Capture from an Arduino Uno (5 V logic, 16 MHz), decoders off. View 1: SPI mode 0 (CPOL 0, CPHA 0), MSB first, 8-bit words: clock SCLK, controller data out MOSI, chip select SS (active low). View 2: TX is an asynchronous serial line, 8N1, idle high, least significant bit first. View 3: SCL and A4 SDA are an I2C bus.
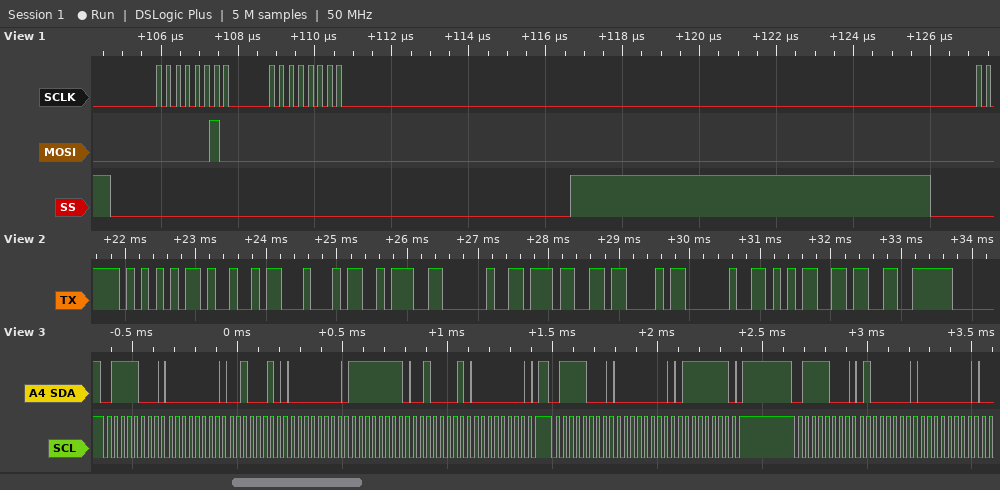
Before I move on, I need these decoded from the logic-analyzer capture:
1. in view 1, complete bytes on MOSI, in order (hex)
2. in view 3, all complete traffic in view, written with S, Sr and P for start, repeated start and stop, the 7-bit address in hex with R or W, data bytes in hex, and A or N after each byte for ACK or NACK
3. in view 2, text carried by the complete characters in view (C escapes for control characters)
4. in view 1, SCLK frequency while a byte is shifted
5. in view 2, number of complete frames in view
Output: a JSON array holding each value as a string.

["0x02 0x00", "S 3CW A 00 A 22 A 00 A FF A 21 A 00 A P S 3CW A 00 A 7F A P S 3CW A 40 A 00 A", "\"UID: 7C 53\"", "4 MHz", "10"]
